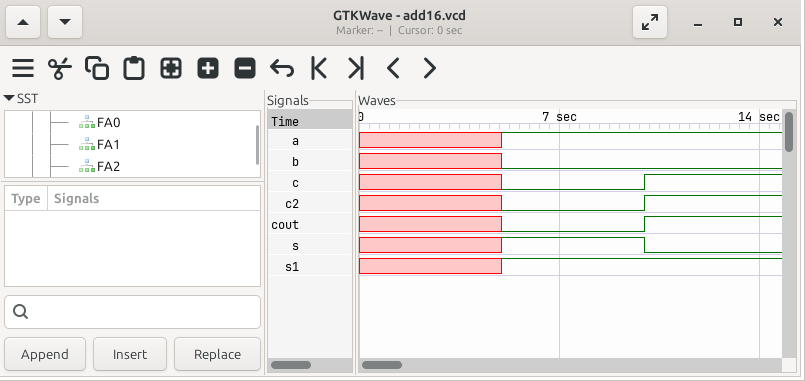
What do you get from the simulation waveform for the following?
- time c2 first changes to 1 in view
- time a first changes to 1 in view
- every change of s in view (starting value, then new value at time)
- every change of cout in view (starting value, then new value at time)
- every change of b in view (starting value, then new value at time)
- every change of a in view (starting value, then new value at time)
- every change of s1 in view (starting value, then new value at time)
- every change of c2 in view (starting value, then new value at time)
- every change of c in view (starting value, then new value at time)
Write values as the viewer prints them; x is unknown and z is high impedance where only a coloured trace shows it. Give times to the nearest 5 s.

10 s
5 s
x, 1 at 5 s, 0 at 10 s
x, 0 at 5 s, 1 at 10 s
x, 0 at 5 s
x, 1 at 5 s
x, 1 at 5 s
x, 0 at 5 s, 1 at 10 s
x, 0 at 5 s, 1 at 10 s
